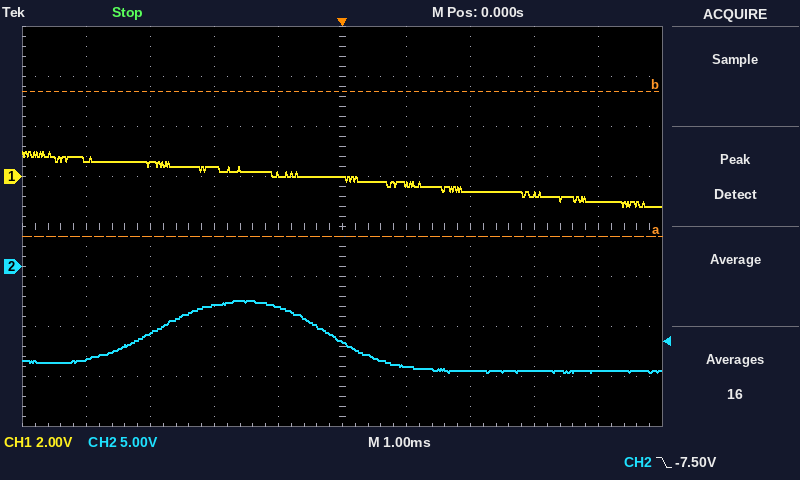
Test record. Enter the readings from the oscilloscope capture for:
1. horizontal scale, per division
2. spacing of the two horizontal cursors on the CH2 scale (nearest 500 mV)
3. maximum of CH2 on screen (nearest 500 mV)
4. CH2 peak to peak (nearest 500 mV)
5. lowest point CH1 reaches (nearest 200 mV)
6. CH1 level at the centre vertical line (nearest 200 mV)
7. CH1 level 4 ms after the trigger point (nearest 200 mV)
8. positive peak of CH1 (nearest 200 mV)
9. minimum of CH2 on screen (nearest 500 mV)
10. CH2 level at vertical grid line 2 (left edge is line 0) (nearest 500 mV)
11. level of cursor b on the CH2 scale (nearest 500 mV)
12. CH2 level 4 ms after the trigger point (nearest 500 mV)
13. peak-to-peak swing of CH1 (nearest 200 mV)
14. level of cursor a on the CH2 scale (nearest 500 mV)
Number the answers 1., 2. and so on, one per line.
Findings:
1. 1 ms
2. 14.5 V
3. -3.5 V
4. 7.0 V
5. -1.2 V
6. 0.0 V
7. -1.0 V
8. 1.0 V
9. -10.5 V
10. -6.5 V
11. 17.5 V
12. -10.5 V
13. 2.2 V
14. 3.0 V
